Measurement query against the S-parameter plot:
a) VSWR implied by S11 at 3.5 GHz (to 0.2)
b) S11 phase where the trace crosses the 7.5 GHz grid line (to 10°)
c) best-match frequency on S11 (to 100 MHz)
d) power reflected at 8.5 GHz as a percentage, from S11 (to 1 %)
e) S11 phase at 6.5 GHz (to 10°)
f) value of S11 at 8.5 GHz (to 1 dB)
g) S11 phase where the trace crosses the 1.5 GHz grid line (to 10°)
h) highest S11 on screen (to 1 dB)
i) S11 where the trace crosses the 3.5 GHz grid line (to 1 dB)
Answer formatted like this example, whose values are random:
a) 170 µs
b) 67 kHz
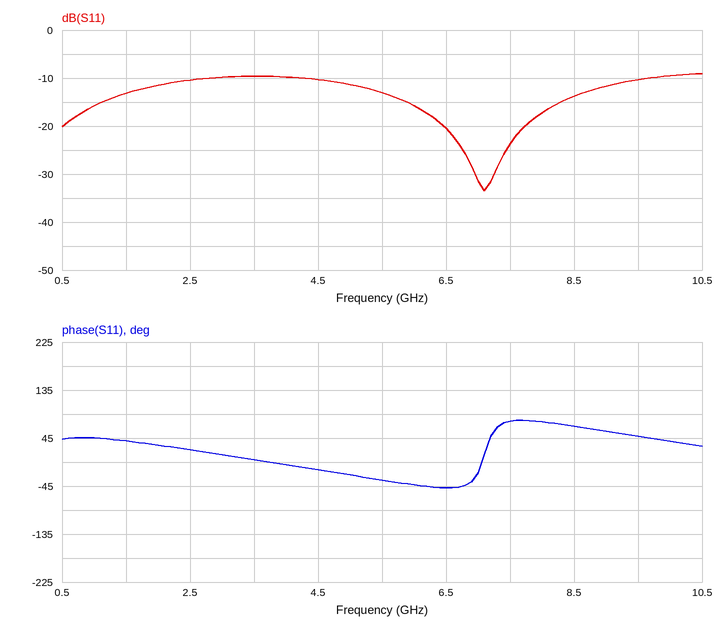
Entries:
a) 2.0
b) 80°
c) 7.1 GHz
d) 4 %
e) -50°
f) -14 dB
g) 40°
h) -9 dB
i) -10 dB
